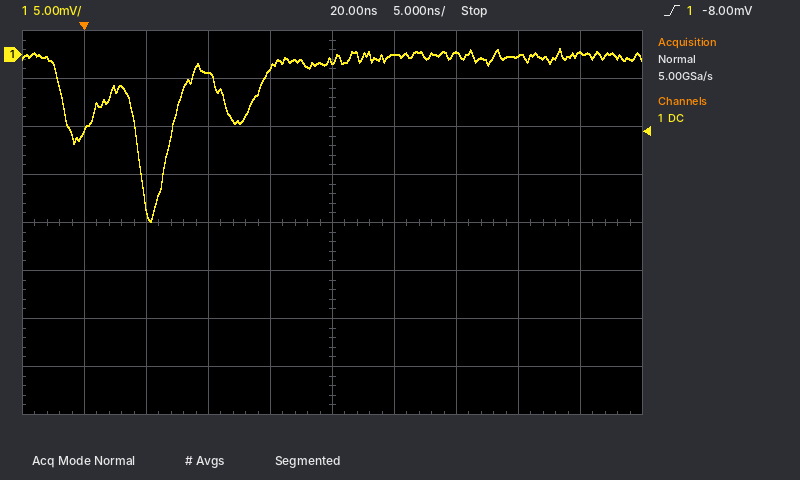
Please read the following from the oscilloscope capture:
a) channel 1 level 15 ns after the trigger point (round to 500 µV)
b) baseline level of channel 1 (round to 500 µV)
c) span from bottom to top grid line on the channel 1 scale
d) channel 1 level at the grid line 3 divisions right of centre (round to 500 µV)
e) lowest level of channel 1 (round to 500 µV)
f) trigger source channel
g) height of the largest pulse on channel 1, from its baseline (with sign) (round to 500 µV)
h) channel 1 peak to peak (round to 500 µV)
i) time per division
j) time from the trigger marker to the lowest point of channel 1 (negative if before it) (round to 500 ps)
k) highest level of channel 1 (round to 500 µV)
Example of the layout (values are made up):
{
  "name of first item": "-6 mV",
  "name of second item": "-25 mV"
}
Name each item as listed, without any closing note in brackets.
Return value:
{
  "channel 1 level 15 ns after the trigger point": "-1.5 mV",
  "baseline level of channel 1": "-500 µV",
  "span from bottom to top grid line on the channel 1 scale": "40 mV",
  "channel 1 level at the grid line 3 divisions right of centre": "0.0 mV",
  "lowest level of channel 1": "-17.5 mV",
  "trigger source channel": "channel 1",
  "height of the largest pulse on channel 1, from its baseline (with sign)": "-17.0 mV",
  "channel 1 peak to peak": "18.0 mV",
  "time per division": "5 ns",
  "time from the trigger marker to the lowest point of channel 1 (negative if before it)": "+5.5 ns",
  "highest level of channel 1": "500 µV"
}
